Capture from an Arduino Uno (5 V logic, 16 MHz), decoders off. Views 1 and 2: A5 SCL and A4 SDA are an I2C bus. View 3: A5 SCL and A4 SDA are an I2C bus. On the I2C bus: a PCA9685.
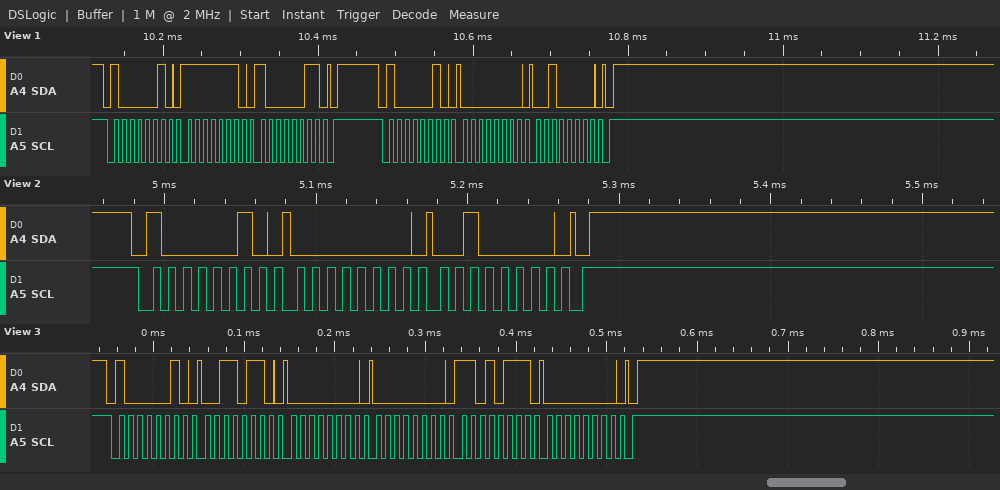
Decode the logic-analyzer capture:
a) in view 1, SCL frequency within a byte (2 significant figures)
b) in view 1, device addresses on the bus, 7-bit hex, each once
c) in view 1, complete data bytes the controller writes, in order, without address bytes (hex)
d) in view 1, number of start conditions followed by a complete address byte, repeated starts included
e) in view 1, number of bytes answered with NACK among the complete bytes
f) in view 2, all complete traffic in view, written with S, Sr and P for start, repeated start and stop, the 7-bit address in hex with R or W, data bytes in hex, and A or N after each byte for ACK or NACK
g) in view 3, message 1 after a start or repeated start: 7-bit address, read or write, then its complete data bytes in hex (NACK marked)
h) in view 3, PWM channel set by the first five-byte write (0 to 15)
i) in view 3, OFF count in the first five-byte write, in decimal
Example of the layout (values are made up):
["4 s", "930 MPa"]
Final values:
["100 kHz", "0x41", "FE 83 00 20", "2", "0", "S 41W A 00 A 20 A P", "0x41 write: 36 00 00 D7 00", "12", "215"]
